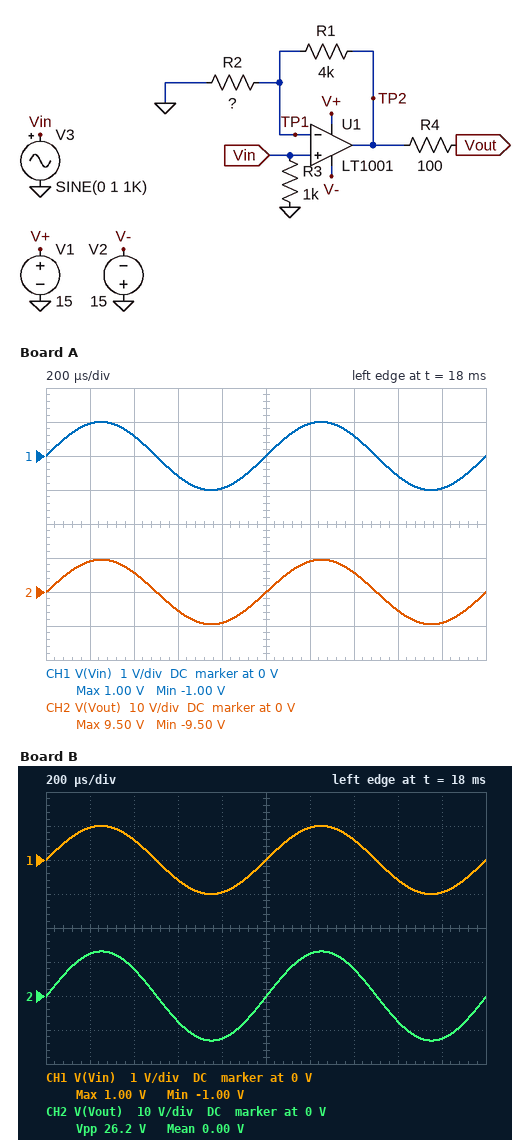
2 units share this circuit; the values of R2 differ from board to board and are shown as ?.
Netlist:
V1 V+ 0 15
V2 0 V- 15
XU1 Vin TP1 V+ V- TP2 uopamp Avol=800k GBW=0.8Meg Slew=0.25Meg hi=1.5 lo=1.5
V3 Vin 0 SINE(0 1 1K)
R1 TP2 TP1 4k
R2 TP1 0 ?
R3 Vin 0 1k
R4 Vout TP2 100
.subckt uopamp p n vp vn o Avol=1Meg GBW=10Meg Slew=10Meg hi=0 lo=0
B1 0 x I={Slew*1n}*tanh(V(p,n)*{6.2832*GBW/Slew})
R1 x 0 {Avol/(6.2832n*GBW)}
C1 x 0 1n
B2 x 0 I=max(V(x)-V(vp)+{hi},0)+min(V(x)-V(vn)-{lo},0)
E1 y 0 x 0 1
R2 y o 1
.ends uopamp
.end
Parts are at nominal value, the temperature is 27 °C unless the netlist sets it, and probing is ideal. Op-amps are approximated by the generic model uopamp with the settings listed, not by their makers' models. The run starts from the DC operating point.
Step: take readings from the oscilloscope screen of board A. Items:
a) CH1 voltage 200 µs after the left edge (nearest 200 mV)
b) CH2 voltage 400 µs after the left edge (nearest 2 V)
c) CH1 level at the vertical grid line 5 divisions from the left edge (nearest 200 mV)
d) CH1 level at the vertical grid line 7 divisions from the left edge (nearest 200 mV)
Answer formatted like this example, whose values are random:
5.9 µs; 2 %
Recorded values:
1.0 V; 6 V; 0 V; 600 mV
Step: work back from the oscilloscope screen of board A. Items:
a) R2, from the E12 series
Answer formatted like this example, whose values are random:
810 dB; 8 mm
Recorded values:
470 Ω
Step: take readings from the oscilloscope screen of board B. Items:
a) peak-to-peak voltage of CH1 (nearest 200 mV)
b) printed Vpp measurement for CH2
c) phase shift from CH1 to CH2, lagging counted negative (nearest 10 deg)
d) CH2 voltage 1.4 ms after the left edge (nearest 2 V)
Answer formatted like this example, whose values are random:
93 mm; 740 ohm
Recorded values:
2.0 V; 26.2 V; 0 deg; 8 V
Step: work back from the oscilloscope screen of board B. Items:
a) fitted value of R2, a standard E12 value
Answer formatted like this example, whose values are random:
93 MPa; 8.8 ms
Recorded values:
330 Ω
